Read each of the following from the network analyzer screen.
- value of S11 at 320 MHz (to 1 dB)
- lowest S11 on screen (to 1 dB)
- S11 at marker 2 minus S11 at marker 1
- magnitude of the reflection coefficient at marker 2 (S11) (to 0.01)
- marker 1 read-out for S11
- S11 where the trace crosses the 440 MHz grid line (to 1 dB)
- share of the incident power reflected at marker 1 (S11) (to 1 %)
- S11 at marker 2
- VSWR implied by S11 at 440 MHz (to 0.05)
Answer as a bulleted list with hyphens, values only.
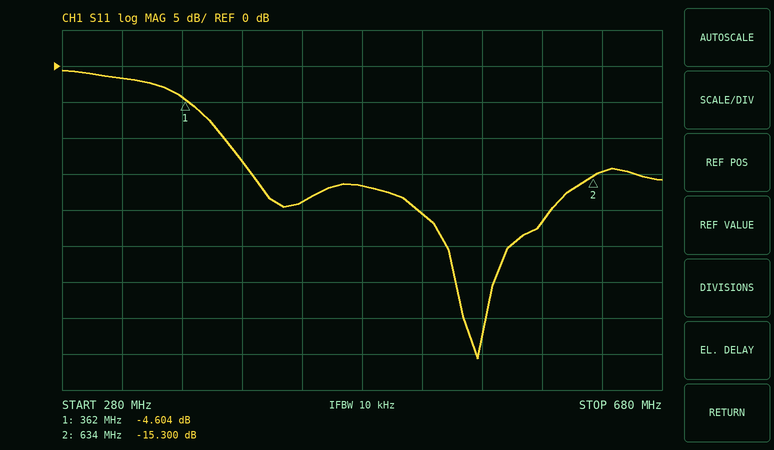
- -2 dB
- -41 dB
- -10.696 dB
- 0.17
- -4.604 dB
- -19 dB
- 35 %
- -15.300 dB
- 1.25
